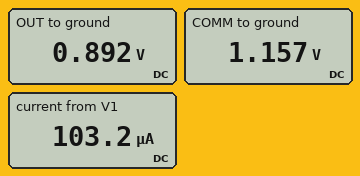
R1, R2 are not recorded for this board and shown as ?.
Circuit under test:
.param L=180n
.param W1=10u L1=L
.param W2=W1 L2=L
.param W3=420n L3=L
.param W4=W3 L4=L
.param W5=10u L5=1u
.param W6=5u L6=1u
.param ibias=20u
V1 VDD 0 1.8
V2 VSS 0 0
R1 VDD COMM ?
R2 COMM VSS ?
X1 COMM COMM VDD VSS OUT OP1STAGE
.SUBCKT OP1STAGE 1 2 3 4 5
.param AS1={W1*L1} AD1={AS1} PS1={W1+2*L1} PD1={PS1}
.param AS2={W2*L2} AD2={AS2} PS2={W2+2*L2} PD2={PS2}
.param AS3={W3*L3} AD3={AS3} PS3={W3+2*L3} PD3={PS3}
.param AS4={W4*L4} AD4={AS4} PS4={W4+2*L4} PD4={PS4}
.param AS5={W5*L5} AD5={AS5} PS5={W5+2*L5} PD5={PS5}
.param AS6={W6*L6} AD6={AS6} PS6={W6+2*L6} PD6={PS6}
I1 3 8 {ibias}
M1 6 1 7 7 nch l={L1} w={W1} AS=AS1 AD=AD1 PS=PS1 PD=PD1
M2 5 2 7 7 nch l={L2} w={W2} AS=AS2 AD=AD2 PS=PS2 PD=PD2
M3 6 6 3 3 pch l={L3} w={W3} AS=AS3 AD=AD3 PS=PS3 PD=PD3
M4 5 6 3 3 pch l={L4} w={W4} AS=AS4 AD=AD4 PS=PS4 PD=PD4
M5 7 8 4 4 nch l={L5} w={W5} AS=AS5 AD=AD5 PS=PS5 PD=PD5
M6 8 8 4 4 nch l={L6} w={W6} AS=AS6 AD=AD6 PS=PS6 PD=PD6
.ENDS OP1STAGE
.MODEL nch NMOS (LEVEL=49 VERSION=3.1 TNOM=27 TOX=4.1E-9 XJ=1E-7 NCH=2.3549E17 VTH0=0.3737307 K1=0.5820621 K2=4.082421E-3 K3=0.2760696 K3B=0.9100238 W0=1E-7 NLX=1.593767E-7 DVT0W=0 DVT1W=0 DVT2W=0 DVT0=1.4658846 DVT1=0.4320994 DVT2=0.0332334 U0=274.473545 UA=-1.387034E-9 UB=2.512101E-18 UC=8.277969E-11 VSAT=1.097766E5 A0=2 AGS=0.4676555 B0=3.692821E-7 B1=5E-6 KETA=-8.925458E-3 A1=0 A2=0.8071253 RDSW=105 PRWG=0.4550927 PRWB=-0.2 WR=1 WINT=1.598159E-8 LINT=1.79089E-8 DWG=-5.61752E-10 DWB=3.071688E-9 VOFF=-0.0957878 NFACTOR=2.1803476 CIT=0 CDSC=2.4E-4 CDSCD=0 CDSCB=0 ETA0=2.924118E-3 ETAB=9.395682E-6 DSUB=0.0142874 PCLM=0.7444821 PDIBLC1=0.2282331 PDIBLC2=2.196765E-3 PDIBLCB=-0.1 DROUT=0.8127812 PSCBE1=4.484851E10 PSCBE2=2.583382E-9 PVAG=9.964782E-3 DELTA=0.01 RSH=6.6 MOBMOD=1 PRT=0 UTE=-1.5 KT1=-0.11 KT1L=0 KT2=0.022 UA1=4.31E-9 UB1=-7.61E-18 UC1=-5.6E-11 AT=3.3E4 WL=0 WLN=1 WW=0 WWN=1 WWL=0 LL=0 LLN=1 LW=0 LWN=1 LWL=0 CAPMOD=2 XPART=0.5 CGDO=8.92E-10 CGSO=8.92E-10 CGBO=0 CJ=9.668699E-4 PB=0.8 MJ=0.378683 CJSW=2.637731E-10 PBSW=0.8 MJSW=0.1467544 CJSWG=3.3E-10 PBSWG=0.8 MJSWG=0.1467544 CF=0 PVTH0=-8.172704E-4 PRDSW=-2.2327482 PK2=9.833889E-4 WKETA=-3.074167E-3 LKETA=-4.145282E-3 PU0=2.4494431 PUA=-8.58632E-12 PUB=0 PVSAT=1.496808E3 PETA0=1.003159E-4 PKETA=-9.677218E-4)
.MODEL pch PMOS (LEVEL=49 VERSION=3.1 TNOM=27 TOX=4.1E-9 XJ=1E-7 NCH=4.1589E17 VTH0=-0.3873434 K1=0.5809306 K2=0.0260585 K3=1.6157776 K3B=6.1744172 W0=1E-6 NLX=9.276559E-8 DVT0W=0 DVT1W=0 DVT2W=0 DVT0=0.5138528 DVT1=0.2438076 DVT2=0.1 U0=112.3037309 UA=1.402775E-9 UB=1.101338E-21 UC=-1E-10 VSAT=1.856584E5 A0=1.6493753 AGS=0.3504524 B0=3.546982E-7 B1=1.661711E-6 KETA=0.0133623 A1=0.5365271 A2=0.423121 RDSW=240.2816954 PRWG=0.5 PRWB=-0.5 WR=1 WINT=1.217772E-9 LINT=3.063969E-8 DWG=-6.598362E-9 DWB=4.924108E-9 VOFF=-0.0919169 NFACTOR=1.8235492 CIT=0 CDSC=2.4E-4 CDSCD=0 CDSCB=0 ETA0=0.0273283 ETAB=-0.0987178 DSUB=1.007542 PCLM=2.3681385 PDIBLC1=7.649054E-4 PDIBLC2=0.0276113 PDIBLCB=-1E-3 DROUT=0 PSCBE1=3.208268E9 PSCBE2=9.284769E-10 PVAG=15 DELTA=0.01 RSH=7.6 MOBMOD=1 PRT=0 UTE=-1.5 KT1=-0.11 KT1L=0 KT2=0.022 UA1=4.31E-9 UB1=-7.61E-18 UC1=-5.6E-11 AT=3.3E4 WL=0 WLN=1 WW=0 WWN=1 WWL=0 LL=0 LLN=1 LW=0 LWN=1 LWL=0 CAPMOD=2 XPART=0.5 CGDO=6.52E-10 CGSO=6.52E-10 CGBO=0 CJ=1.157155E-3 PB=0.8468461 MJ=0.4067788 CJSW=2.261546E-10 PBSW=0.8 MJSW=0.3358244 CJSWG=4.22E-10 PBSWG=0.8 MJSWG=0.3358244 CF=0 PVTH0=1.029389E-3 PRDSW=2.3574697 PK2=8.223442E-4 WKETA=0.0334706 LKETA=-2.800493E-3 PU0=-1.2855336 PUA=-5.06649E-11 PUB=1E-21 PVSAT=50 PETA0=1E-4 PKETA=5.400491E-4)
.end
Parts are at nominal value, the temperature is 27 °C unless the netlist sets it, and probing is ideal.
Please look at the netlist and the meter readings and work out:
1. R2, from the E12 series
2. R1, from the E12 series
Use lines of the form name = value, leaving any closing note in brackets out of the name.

R2, from the E12 series = 27 kΩ
R1, from the E12 series = 15 kΩ
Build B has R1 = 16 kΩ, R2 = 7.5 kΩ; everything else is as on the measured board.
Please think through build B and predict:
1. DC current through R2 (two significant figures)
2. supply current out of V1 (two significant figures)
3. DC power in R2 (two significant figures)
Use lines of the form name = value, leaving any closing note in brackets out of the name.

DC current through R2 = 77 µA
supply current out of V1 = 130 µA
DC power in R2 = 44 µW
